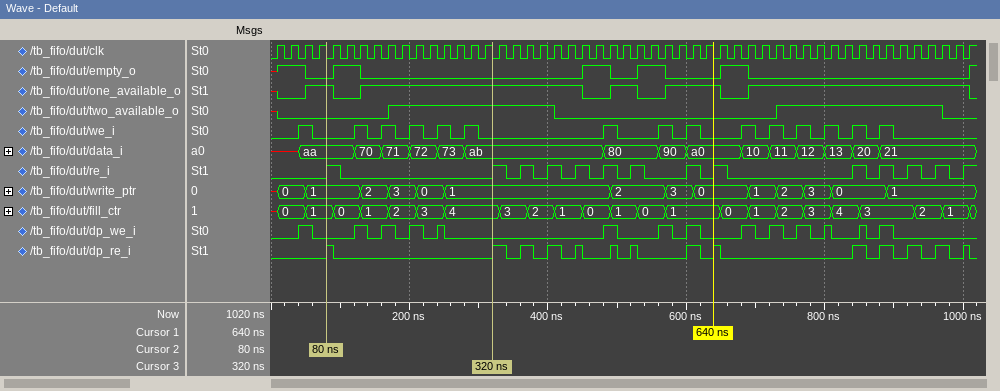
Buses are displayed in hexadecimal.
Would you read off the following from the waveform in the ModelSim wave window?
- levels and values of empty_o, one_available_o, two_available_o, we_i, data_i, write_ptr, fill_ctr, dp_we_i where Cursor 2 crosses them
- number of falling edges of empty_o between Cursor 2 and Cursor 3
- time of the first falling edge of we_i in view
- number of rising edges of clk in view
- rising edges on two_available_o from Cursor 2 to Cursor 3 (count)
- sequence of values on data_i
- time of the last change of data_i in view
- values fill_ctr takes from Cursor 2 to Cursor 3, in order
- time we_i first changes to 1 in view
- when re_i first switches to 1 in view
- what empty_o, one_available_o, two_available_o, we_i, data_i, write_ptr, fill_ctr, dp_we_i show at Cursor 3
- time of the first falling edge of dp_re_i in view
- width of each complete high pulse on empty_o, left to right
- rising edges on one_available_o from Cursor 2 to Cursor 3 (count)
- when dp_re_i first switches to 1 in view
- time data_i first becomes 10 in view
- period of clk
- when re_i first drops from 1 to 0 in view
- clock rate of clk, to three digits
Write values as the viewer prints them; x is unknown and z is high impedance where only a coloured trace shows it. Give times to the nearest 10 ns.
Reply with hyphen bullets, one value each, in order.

- empty_o=0, one_available_o=1, two_available_o=0, we_i=0, data_i=aa, write_ptr=1, fill_ctr=1, dp_we_i=0
- 1
- 60 ns
- 51
- 1
- x, aa, 70, 71, 72, 73, ab, 80, 90, a0, 10, 11, 12, 13, 20, 21
- 880 ns
- 1, 0, 1, 2, 3, 4
- 40 ns
- 80 ns
- empty_o=0, one_available_o=1, two_available_o=1, we_i=0, data_i=ab, write_ptr=1, fill_ctr=4, dp_we_i=0
- 90 ns
- 40 ns, 40 ns, 40 ns, 40 ns
- 1
- 80 ns
- 680 ns
- 20 ns
- 100 ns
- 50.0 MHz
